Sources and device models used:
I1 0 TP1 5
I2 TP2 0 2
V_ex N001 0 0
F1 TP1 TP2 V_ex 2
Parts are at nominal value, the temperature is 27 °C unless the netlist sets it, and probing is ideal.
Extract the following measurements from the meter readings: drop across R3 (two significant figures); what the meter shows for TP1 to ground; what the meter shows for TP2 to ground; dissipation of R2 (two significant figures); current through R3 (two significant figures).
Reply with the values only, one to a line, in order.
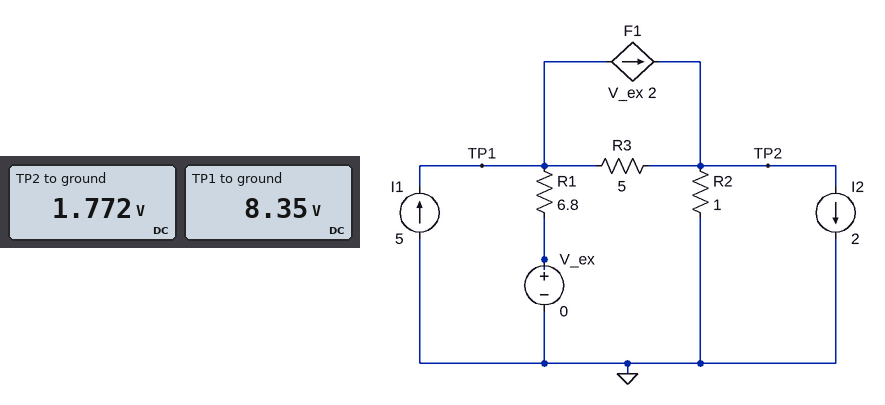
6.6 V
8.35 V
1.772 V
3.1 W
1.3 A
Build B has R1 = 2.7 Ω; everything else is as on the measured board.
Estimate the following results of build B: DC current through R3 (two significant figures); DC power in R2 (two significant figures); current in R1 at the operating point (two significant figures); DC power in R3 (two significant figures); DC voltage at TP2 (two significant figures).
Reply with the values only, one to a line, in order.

510 mA
2.3 W
1.5 A
1.3 W
1.5 V
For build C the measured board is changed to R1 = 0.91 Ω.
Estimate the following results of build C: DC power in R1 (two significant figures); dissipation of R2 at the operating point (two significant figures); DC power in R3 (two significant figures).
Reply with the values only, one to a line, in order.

2.5 W
1.8 W
5.3 mW
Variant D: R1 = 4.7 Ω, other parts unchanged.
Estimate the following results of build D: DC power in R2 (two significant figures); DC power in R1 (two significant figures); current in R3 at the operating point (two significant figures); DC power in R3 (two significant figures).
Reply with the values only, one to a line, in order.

2.7 W
8.6 W
940 mA
4.4 W
